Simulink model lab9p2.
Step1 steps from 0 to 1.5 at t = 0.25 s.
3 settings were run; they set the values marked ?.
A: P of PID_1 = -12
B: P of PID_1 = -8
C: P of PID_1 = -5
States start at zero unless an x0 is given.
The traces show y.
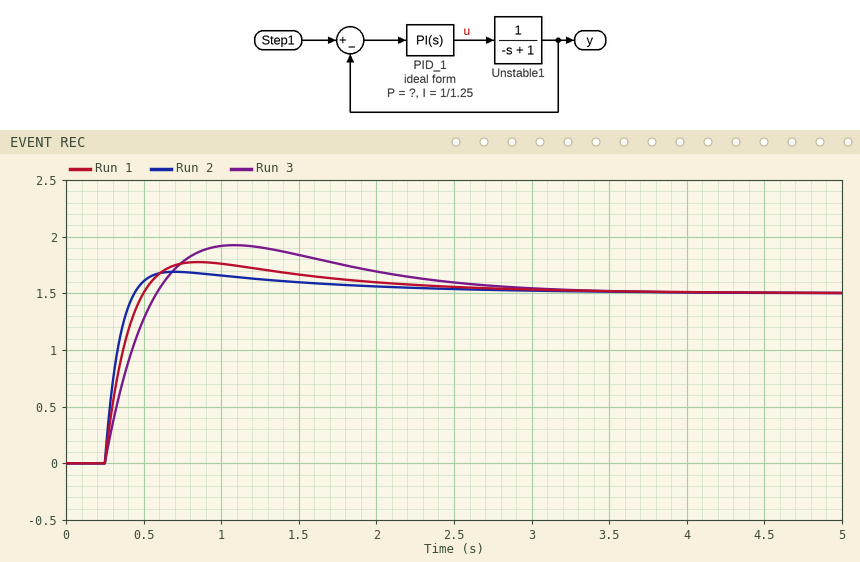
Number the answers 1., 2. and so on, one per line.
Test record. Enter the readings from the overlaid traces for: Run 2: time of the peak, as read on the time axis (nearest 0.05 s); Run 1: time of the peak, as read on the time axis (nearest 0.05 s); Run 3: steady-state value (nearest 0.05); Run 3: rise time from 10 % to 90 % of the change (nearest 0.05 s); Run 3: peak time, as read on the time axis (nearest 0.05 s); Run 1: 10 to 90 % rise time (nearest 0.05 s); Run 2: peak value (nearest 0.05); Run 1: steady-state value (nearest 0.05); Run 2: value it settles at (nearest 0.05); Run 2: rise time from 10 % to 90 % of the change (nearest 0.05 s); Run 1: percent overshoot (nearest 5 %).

1. 0.70 s
2. 0.85 s
3. 1.50
4. 0.25 s
5. 1.10 s
6. 0.20 s
7. 1.70
8. 1.50
9. 1.50
10. 0.15 s
11. 20 %
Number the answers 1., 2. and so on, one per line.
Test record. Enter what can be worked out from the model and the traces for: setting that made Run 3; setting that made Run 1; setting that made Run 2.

1. C
2. B
3. A
